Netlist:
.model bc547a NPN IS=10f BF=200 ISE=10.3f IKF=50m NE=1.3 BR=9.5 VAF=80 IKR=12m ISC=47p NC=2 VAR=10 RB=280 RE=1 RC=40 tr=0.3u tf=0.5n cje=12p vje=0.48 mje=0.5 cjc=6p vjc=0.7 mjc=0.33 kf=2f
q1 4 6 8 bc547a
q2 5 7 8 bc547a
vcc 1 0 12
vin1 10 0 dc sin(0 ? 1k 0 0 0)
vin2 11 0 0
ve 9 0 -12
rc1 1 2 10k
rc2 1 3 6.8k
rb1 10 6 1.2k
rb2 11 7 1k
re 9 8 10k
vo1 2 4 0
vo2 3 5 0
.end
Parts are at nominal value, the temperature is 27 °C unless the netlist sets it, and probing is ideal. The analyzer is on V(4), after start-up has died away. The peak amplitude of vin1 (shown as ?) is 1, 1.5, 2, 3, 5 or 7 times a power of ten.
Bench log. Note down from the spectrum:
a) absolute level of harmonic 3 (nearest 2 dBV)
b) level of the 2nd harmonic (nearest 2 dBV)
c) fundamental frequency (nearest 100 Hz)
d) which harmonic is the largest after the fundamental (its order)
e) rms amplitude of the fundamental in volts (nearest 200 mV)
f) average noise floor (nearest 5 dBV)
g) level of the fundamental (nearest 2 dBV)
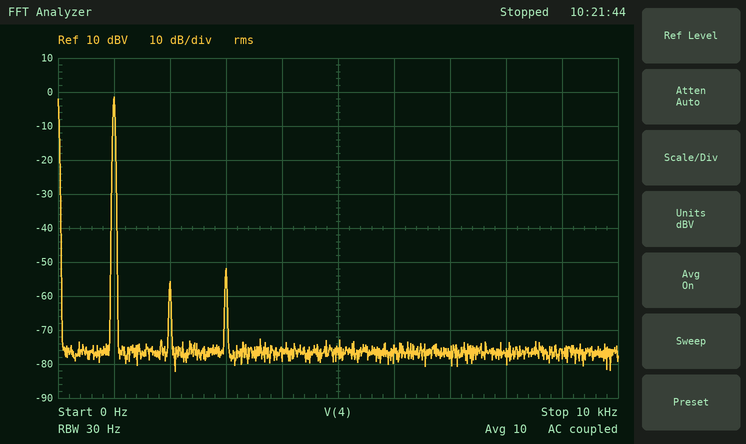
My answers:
-52 dBV
-56 dBV
1.0 kHz
3
800 mV
-75 dBV
-2 dBV
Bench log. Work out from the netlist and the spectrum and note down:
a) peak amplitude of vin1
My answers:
15 mV
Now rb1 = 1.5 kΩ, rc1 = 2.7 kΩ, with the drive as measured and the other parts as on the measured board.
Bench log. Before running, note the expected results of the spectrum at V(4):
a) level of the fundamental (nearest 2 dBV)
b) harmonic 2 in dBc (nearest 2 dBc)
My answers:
-12 dBV
-52 dBc
